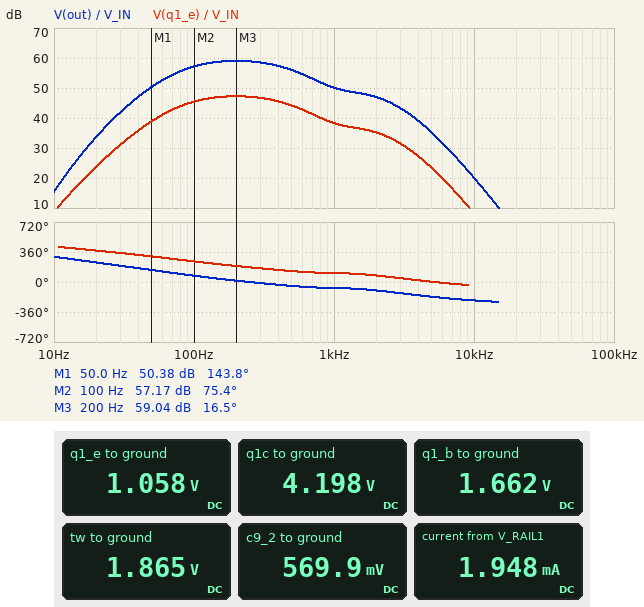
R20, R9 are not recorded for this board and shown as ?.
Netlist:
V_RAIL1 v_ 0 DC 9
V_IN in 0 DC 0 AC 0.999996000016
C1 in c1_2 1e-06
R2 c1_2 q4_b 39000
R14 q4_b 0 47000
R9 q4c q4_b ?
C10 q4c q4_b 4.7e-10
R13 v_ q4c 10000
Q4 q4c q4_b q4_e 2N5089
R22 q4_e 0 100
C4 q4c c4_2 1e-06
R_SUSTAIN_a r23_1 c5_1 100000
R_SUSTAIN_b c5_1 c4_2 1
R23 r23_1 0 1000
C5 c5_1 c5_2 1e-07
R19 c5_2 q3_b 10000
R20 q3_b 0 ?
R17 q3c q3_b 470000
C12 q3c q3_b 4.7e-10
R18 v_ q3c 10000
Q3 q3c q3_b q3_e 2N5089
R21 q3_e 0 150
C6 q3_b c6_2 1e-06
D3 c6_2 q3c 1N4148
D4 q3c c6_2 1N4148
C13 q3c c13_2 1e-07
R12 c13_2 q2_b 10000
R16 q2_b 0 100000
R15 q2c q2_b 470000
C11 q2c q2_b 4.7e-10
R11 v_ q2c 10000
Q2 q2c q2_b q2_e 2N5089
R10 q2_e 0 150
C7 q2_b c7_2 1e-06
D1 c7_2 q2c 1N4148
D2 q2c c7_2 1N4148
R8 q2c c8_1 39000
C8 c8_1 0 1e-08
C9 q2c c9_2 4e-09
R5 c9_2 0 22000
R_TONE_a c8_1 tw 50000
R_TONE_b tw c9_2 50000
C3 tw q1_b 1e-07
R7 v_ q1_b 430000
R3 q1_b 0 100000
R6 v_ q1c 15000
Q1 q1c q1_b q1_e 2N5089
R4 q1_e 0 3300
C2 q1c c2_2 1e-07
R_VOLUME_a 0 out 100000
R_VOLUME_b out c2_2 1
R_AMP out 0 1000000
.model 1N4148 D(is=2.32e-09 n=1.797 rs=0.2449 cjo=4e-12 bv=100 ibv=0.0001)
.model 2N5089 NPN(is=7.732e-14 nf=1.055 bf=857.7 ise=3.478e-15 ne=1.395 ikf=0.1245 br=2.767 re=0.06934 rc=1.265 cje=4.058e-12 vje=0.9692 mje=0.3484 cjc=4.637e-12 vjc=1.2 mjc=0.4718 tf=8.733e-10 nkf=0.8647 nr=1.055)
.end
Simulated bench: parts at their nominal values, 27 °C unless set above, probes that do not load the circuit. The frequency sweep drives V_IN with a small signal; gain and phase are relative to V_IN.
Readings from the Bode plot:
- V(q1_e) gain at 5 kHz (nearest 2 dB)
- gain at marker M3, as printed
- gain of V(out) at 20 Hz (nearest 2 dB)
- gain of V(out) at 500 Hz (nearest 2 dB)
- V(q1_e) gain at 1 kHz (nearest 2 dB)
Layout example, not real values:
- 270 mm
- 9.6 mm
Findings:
- 24 dB
- 59.04 dB
- 34 dB
- 56 dB
- 38 dB
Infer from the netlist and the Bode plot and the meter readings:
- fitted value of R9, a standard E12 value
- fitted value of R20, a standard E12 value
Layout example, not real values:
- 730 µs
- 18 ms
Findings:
- 150 kΩ
- 120 kΩ
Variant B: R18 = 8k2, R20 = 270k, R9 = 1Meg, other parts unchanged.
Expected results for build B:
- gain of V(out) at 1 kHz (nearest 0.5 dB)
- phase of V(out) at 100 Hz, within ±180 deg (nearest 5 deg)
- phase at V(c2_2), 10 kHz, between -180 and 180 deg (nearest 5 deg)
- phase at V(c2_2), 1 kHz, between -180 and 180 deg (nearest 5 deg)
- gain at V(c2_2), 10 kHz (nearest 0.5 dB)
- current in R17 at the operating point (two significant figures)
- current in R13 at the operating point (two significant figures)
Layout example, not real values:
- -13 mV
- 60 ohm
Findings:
- 7.0 dB
- 65 deg
- 95 deg
- -90 deg
- -2.0 dB
- 3.8 µA
- 8.7 µA
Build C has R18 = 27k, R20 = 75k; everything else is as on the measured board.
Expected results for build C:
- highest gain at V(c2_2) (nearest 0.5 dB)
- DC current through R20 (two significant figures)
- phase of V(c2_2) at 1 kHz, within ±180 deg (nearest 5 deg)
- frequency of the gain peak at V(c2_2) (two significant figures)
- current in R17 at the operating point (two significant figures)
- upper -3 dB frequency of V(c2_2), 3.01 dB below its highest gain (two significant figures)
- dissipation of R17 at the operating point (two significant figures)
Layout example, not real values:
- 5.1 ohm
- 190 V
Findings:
- 59.5 dB
- 8.1 µA
- -75 deg
- 190 Hz
- 8.3 µA
- 480 Hz
- 33 µW
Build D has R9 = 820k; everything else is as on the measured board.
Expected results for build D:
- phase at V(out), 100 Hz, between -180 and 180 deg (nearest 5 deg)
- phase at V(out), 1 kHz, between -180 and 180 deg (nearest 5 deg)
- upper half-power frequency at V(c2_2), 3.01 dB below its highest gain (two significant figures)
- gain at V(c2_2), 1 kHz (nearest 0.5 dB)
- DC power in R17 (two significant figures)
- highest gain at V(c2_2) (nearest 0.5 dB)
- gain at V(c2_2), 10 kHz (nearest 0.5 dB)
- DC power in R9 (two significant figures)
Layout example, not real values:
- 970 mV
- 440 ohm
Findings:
- 65 deg
- -65 deg
- 480 Hz
- 32.5 dB
- 20 µW
- 41.5 dB
- 8.5 dB
- 86 µW
